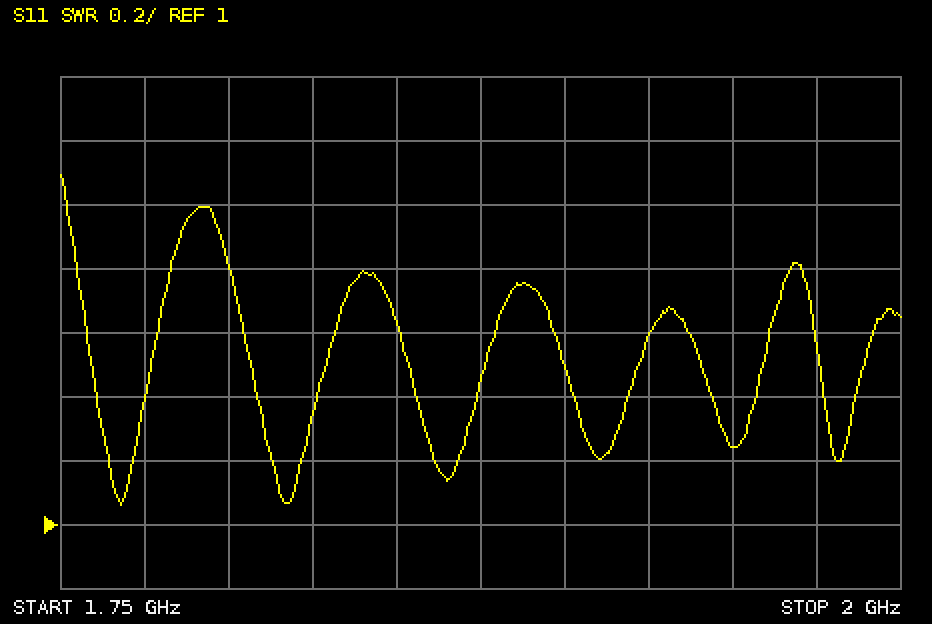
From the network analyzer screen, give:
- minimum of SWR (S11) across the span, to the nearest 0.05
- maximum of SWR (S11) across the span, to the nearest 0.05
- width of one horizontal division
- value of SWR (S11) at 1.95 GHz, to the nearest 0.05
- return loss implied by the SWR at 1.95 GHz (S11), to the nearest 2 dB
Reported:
1.05
2.10
25 MHz
1.25
20 dB
